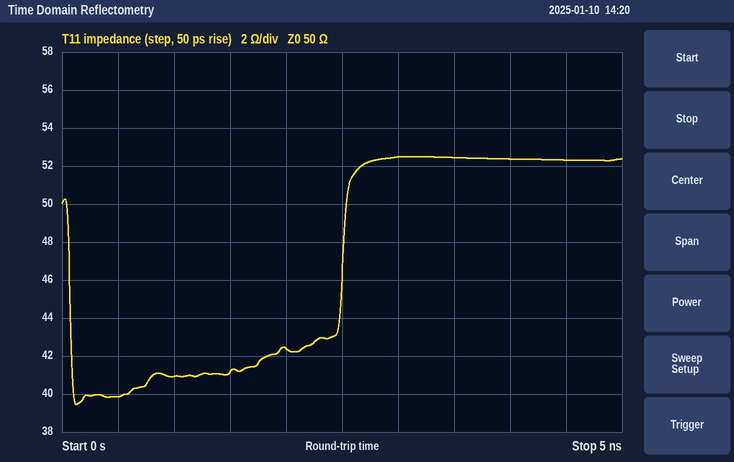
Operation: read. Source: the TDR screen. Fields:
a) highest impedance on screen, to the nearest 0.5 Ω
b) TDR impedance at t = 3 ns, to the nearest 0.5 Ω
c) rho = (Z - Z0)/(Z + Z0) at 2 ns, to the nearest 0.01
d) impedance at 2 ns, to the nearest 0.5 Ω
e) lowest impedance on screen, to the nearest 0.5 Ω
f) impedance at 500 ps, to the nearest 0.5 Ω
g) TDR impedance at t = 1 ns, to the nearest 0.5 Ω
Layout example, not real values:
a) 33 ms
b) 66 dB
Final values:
a) 52.5 Ω
b) 52.5 Ω
c) -0.08
d) 42.5 Ω
e) 39.5 Ω
f) 40.0 Ω
g) 41.0 Ω
